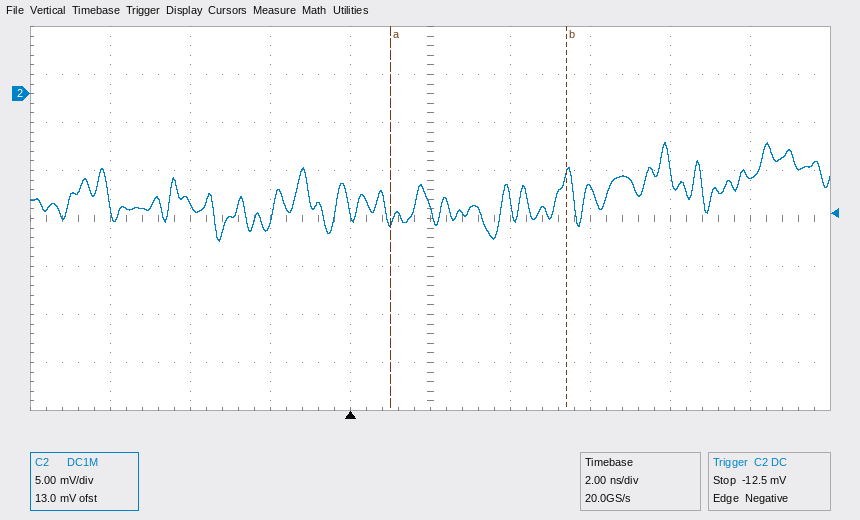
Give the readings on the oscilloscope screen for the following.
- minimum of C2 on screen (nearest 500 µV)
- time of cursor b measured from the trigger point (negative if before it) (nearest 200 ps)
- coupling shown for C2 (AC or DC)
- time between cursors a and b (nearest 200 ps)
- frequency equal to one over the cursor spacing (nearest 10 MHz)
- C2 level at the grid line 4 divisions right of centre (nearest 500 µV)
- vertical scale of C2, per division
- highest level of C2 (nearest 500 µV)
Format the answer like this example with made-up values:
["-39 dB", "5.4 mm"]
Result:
["-15.5 mV", "+5.4 ns", "DC", "4.4 ns", "230 MHz", "-8.5 mV", "5 mV", "-5.0 mV"]
